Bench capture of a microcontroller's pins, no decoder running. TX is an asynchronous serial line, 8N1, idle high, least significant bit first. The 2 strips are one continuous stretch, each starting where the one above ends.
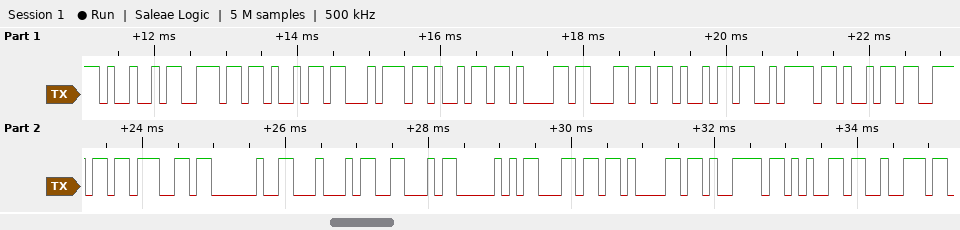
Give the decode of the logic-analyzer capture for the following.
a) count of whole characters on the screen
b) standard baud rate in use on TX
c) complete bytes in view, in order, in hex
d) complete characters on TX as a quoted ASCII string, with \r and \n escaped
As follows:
21
9600 baud
49 6E 69 74 69 61 6C 69 7A 69 6E 67 20 44 46 50 6C 61 79 65 72
"Initializing DFPlayer"
